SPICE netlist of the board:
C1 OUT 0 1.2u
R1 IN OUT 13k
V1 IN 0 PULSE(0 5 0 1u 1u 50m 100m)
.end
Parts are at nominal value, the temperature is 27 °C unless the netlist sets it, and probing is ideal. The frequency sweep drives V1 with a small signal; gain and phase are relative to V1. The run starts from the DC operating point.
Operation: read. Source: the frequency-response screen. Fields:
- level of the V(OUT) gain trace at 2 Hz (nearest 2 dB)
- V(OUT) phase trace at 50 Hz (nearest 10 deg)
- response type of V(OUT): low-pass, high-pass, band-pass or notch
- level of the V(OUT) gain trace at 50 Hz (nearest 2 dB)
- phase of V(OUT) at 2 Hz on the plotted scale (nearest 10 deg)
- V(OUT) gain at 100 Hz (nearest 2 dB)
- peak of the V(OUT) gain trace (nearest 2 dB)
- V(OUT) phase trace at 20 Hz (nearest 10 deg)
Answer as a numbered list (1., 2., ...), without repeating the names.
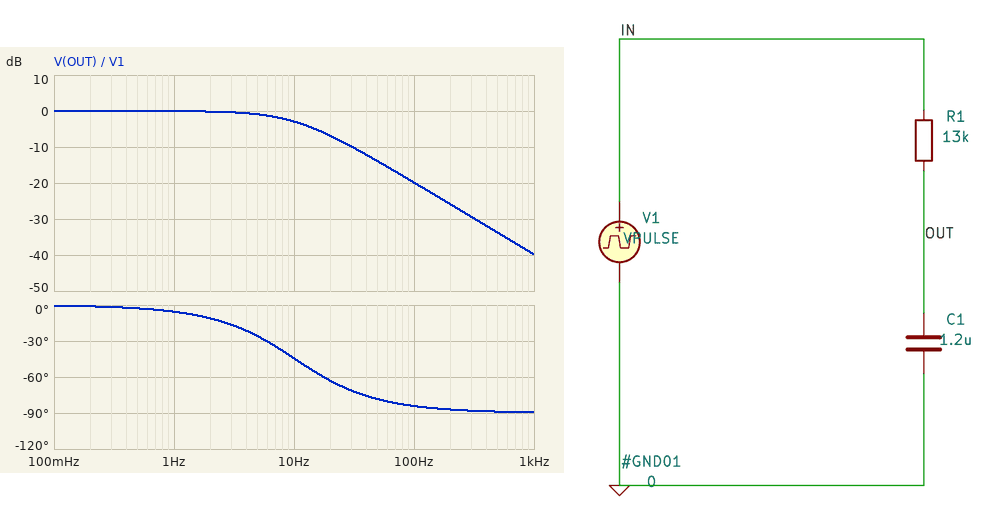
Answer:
1. 0 dB
2. -80 deg
3. low-pass
4. -14 dB
5. -10 deg
6. -20 dB
7. 0 dB
8. -60 deg
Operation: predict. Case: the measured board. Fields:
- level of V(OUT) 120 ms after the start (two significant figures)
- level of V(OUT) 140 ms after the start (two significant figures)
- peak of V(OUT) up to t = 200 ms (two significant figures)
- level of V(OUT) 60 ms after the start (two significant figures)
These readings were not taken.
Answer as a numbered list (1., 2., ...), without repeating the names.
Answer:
1. 3.7 V
2. 4.6 V
3. 4.8 V
4. 2.5 V
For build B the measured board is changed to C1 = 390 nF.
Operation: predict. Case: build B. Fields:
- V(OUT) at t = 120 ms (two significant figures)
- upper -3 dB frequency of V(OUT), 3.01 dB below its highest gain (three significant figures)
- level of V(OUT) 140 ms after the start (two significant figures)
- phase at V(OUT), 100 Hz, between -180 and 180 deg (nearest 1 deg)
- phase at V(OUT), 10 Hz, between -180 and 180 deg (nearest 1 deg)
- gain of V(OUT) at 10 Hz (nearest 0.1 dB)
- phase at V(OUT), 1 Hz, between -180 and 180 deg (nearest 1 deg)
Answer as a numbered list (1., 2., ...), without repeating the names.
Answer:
1. 4.9 V
2. 31.4 Hz
3. 5.0 V
4. -73 deg
5. -18 deg
6. -0.4 dB
7. -2 deg
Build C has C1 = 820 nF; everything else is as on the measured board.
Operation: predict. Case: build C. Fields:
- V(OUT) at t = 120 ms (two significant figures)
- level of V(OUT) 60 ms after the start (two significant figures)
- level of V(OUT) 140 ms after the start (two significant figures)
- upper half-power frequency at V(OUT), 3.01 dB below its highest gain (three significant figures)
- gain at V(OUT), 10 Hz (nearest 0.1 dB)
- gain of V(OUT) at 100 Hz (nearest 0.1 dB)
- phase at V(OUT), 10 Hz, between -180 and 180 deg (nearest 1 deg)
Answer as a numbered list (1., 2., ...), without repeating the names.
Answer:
1. 4.2 V
2. 1.9 V
3. 4.9 V
4. 14.9 Hz
5. -1.6 dB
6. -16.6 dB
7. -34 deg
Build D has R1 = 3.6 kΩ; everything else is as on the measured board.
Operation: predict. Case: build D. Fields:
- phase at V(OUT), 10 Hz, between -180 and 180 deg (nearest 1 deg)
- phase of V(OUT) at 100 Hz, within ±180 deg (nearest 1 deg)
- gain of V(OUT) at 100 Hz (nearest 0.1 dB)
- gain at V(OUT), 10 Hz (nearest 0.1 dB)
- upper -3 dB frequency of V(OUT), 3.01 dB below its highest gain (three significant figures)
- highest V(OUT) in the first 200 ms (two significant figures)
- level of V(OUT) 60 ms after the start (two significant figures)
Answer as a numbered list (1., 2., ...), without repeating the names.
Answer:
1. -15 deg
2. -70 deg
3. -9.2 dB
4. -0.3 dB
5. 36.8 Hz
6. 5.0 V
7. 490 mV
